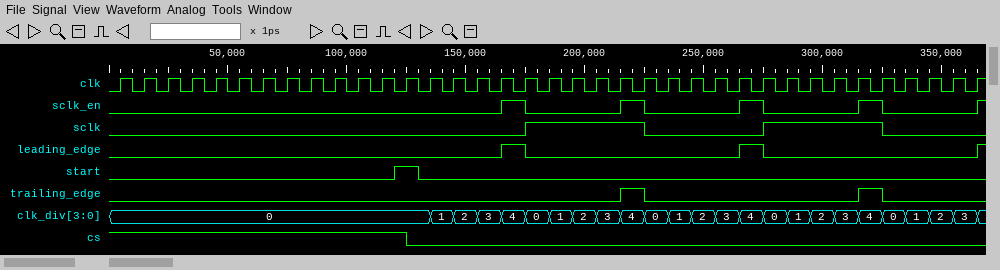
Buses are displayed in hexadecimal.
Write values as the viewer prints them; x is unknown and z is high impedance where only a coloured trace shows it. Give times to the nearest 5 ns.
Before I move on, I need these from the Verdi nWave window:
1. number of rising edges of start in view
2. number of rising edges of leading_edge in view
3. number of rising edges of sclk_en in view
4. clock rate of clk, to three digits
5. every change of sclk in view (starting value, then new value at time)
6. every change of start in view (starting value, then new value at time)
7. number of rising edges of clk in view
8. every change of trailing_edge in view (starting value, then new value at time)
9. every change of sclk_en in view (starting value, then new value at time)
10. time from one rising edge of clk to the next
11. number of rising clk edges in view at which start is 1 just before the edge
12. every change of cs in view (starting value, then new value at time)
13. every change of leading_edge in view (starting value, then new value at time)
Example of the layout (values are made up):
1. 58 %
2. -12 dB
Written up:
1. 1
2. 3
3. 5
4. 100 MHz
5. 0, 1 at 175 ns, 0 at 225 ns, 1 at 275 ns, 0 at 325 ns
6. 0, 1 at 120 ns, 0 at 130 ns
7. 37
8. 0, 1 at 215 ns, 0 at 225 ns, 1 at 315 ns, 0 at 325 ns
9. 0, 1 at 165 ns, 0 at 175 ns, 1 at 215 ns, 0 at 225 ns, 1 at 265 ns, 0 at 275 ns, 1 at 315 ns, 0 at 325 ns, 1 at 365 ns
10. 10 ns
11. 1
12. 1, 0 at 125 ns
13. 0, 1 at 165 ns, 0 at 175 ns, 1 at 265 ns, 0 at 275 ns, 1 at 365 ns
